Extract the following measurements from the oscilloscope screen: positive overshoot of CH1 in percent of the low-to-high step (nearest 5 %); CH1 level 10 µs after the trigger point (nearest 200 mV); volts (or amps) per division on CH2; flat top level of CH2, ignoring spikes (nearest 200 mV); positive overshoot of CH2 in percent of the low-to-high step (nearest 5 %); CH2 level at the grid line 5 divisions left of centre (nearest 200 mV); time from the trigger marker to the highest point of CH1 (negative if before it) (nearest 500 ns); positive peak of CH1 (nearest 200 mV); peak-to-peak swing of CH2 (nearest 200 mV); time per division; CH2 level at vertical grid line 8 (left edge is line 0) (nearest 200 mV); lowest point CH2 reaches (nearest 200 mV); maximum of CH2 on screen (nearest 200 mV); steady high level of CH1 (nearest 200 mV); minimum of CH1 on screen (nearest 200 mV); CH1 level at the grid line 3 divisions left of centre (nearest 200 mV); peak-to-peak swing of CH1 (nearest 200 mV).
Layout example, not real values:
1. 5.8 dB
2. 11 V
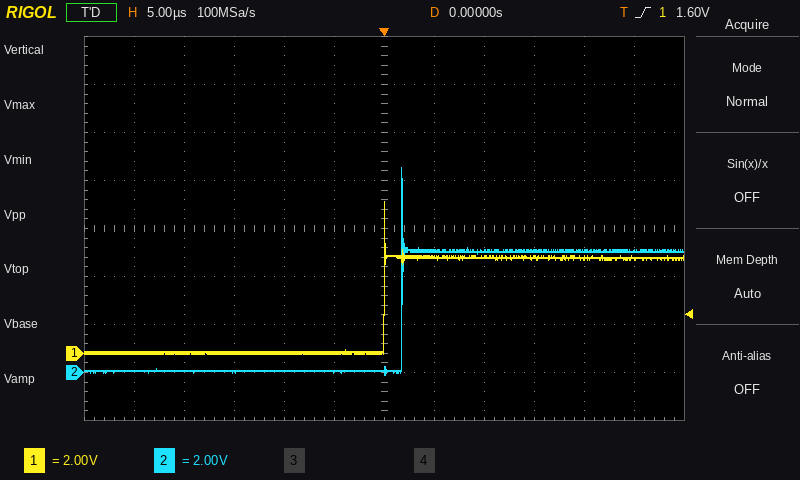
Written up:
1. 60 %
2. 4.0 V
3. 2 V
4. 5.0 V
5. 70 %
6. 0.0 V
7. 0.0 µs
8. 6.4 V
9. 8.6 V
10. 5 µs
11. 5.0 V
12. 0.0 V
13. 8.6 V
14. 4.0 V
15. 0.0 V
16. 0.0 V
17. 6.4 V
